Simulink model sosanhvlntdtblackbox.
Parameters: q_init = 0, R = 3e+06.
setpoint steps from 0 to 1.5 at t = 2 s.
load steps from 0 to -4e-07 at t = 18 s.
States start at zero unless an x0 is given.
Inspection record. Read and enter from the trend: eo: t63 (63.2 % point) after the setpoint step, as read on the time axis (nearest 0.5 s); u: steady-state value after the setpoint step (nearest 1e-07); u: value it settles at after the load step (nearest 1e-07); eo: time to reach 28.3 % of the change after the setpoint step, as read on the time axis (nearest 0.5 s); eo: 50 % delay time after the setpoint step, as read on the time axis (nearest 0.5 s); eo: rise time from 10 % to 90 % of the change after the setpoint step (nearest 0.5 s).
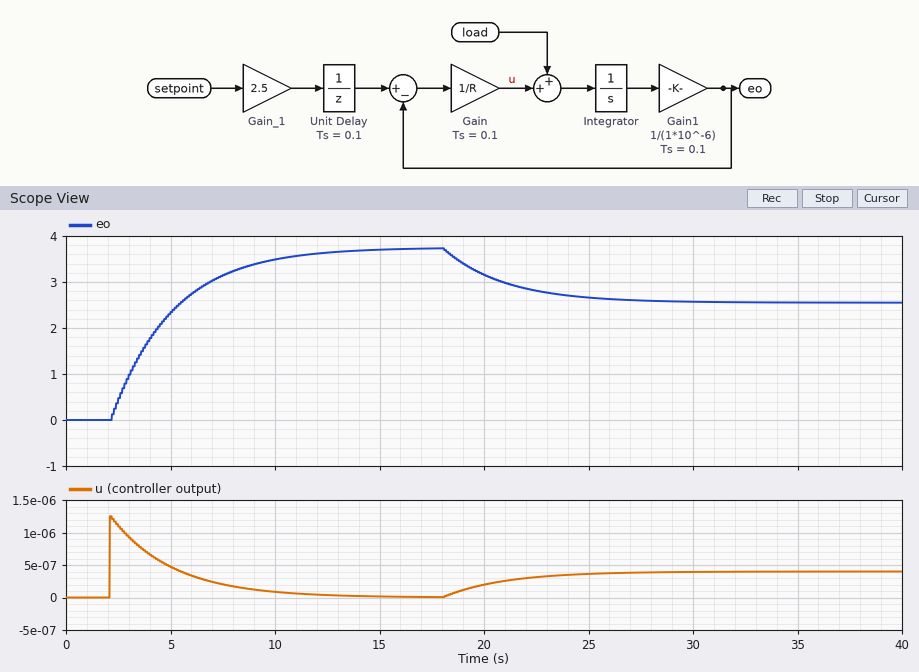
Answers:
5.0 s
0.0000000
0.0000004
3.0 s
4.0 s
6.5 s
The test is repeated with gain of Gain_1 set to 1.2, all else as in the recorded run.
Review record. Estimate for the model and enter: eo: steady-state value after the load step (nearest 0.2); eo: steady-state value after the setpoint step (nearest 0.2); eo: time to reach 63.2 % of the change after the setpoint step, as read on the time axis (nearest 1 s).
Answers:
0.6
1.8
5 s
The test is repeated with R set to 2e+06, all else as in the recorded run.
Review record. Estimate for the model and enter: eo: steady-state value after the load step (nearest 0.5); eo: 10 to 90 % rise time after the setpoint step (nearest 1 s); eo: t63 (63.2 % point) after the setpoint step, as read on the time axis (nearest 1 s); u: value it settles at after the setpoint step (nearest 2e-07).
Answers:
3.0
4 s
4 s
0.0000000
